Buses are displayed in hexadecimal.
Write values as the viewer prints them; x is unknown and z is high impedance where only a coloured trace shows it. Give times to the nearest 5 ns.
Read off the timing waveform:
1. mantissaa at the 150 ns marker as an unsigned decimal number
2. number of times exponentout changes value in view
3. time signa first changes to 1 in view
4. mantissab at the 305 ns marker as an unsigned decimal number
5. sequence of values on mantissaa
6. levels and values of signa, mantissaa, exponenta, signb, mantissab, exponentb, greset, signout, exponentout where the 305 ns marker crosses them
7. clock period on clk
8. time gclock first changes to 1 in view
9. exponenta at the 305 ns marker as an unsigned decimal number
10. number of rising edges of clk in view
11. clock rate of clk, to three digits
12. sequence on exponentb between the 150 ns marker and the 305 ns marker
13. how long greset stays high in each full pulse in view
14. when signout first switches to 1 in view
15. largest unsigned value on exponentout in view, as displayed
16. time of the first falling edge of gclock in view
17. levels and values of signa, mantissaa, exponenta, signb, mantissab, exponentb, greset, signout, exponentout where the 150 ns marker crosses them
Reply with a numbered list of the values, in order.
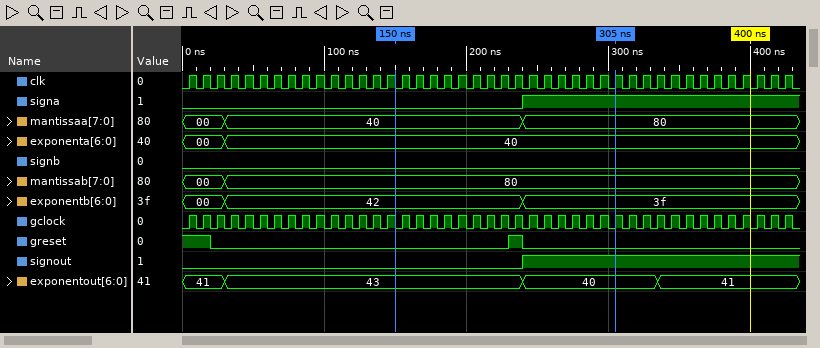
1. 64
2. 3
3. 240 ns
4. 128
5. 00, 40, 80
6. signa=1, mantissaa=80, exponenta=40, signb=0, mantissab=80, exponentb=3f, greset=0, signout=1, exponentout=40
7. 10 ns
8. 5 ns
9. 64
10. 43
11. 100 MHz
12. 42, 3f
13. 10 ns
14. 240 ns
15. 43
16. 10 ns
17. signa=0, mantissaa=40, exponenta=40, signb=0, mantissab=80, exponentb=42, greset=0, signout=0, exponentout=43
